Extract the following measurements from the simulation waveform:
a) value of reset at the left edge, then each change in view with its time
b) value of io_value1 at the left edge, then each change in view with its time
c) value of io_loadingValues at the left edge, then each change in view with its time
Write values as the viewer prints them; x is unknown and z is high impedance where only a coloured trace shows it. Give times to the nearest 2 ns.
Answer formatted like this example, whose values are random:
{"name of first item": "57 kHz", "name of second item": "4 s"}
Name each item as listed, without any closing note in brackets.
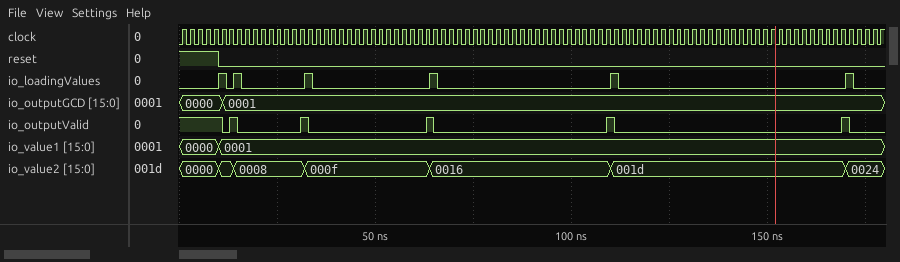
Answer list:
{"value of reset at the left edge, then each change in view with its time": "1, 0 at 10 ns", "value of io_value1 at the left edge, then each change in view with its time": "0000, 0001 at 10 ns", "value of io_loadingValues at the left edge, then each change in view with its time": "0, 1 at 10 ns, 0 at 12 ns, 1 at 14 ns, 0 at 16 ns, 1 at 32 ns, 0 at 34 ns, 1 at 64 ns, 0 at 66 ns, 1 at 110 ns, 0 at 112 ns, 1 at 170 ns, 0 at 172 ns"}
